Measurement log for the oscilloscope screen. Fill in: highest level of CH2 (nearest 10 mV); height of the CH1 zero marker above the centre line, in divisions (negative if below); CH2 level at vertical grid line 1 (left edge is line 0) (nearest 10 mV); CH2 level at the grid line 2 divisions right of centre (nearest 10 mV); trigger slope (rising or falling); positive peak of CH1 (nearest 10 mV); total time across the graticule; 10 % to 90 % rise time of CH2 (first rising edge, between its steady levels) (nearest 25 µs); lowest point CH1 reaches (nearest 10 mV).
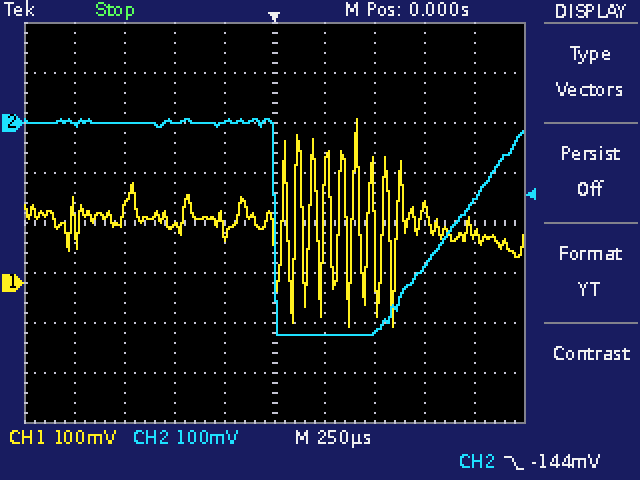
10 mV
-1.2 div
0 mV
-420 mV
falling
330 mV
2.5 ms
625 µs
-90 mV
